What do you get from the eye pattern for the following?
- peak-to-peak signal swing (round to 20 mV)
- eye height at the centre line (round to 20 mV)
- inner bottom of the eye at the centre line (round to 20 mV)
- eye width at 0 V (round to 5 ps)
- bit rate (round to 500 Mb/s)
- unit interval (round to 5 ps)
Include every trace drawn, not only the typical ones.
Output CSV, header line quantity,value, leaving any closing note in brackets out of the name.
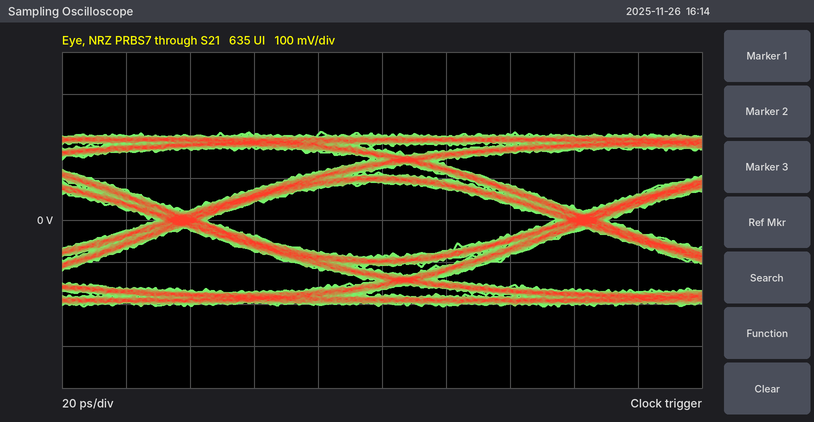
quantity,value
peak-to-peak signal swing,420 mV
eye height at the centre line,180 mV
inner bottom of the eye at the centre line,-80 mV
eye width at 0 V,110 ps
bit rate,8.0 Gb/s
unit interval,125 ps
